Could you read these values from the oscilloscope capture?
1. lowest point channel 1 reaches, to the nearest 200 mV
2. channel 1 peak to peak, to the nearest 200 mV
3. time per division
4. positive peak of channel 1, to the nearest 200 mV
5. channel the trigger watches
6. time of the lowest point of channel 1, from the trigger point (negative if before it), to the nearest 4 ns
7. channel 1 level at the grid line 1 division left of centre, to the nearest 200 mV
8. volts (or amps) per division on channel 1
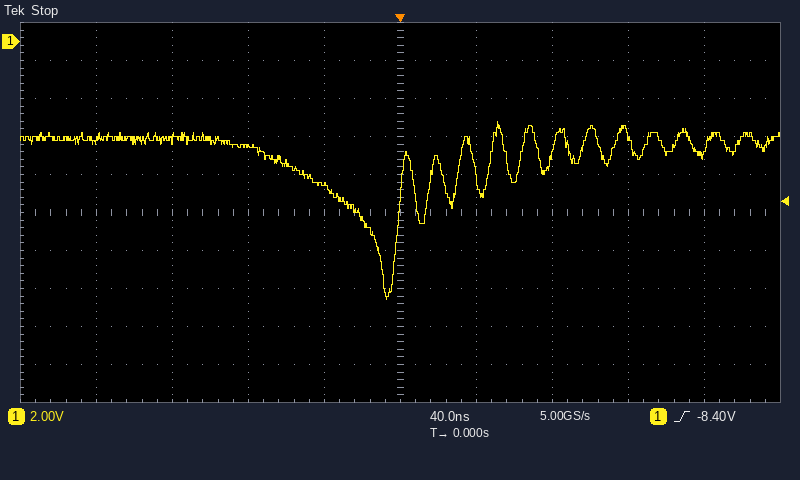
-13.6 V
9.4 V
40 ns
-4.2 V
channel 1
-8 ns
-7.6 V
2 V
